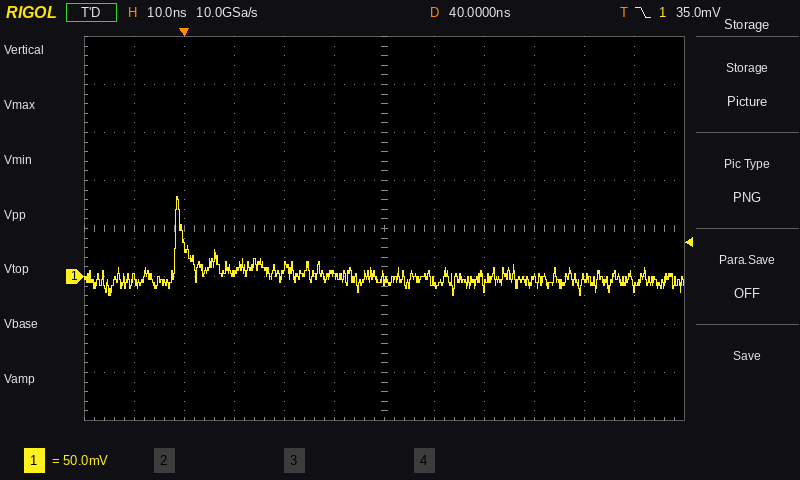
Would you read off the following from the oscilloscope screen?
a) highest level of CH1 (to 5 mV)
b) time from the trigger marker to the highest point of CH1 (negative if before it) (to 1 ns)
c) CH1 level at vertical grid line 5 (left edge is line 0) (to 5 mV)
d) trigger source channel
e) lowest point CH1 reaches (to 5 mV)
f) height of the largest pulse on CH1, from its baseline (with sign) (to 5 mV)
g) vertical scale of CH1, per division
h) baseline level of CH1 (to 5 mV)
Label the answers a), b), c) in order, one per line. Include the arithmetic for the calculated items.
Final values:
a) 85 mV
b) -1 ns
c) 0 mV
d) CH1
e) -20 mV
f) 85 mV − (0 mV) = +85 mV
g) 50 mV
h) 0 mV
